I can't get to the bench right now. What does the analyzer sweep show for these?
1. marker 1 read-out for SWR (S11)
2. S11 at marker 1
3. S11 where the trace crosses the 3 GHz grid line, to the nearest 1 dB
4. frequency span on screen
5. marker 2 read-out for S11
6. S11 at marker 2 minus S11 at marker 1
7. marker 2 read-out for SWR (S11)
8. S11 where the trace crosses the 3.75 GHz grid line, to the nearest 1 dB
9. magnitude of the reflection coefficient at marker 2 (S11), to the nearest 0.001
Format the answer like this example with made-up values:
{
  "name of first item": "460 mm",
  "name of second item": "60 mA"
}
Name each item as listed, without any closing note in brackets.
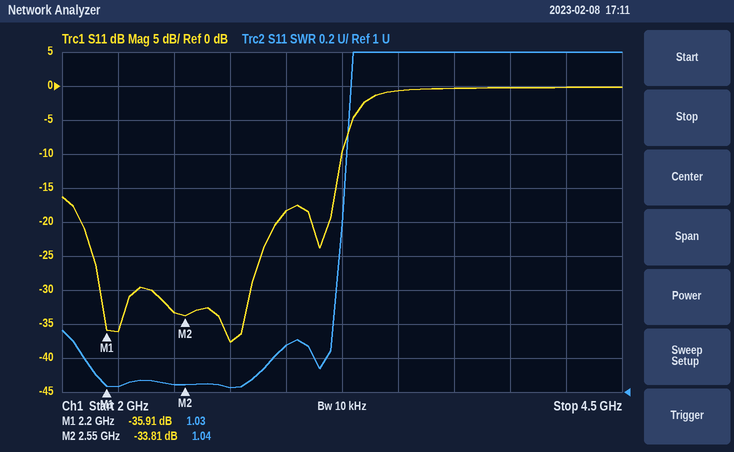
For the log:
{
  "marker 1 read-out for SWR": "1.03",
  "S11 at marker 1": "-35.91 dB",
  "S11 where the trace crosses the 3 GHz grid line, to the nearest 1 dB": "-18 dB",
  "frequency span on screen": "2.5 GHz",
  "marker 2 read-out for S11": "-33.81 dB",
  "S11 at marker 2 minus S11 at marker 1": "2.10 dB",
  "marker 2 read-out for SWR": "1.04",
  "S11 where the trace crosses the 3.75 GHz grid line, to the nearest 1 dB": "0 dB",
  "magnitude of the reflection coefficient at marker 2 (S11), to the nearest 0.001": "0.020"
}
